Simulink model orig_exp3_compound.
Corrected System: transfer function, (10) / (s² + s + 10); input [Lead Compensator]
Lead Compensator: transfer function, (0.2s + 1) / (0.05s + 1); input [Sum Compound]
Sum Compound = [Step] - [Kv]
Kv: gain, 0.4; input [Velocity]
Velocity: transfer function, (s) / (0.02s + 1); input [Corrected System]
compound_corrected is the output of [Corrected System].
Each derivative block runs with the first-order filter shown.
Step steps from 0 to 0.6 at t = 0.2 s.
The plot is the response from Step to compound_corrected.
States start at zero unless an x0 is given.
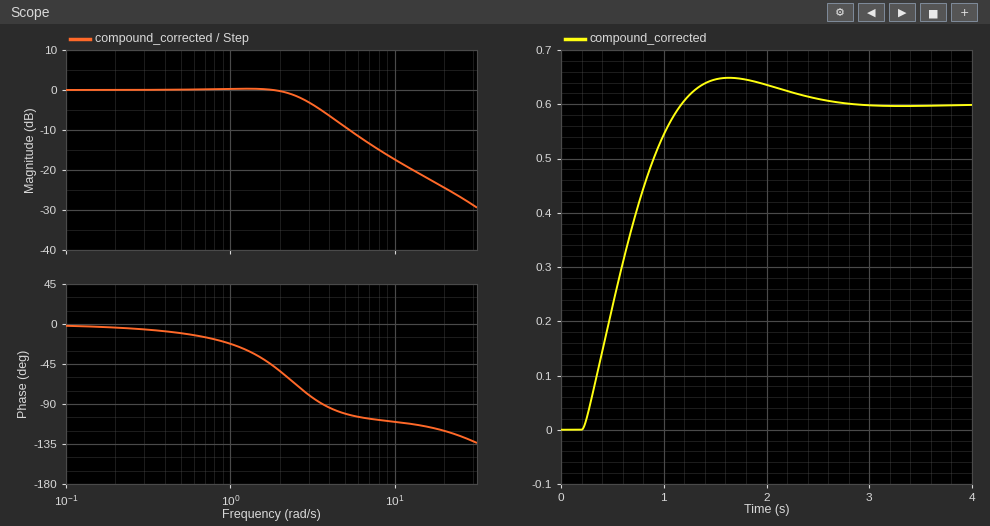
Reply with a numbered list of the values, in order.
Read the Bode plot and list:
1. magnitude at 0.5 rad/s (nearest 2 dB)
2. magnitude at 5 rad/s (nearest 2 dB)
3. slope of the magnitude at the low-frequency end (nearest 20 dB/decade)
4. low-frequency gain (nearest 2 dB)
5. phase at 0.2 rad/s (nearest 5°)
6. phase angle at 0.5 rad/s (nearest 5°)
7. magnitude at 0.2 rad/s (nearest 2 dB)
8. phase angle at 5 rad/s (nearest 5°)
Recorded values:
1. 0 dB
2. -10 dB
3. 0 dB/decade
4. 0 dB
5. -5°
6. -10°
7. 0 dB
8. -100°
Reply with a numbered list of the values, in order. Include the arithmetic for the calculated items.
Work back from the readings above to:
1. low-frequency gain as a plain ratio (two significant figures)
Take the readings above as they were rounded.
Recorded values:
1. 10^(0 / 20) = 1.0
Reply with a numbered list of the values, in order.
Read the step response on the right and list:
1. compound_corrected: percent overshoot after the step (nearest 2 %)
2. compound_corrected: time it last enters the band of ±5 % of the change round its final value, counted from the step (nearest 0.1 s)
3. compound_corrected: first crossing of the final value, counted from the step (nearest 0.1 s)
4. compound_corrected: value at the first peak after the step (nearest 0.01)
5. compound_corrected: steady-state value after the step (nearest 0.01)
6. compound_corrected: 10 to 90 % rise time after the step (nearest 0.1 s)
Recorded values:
1. 8 %
2. 1.9 s
3. 1.0 s
4. 0.65
5. 0.60
6. 0.7 s
